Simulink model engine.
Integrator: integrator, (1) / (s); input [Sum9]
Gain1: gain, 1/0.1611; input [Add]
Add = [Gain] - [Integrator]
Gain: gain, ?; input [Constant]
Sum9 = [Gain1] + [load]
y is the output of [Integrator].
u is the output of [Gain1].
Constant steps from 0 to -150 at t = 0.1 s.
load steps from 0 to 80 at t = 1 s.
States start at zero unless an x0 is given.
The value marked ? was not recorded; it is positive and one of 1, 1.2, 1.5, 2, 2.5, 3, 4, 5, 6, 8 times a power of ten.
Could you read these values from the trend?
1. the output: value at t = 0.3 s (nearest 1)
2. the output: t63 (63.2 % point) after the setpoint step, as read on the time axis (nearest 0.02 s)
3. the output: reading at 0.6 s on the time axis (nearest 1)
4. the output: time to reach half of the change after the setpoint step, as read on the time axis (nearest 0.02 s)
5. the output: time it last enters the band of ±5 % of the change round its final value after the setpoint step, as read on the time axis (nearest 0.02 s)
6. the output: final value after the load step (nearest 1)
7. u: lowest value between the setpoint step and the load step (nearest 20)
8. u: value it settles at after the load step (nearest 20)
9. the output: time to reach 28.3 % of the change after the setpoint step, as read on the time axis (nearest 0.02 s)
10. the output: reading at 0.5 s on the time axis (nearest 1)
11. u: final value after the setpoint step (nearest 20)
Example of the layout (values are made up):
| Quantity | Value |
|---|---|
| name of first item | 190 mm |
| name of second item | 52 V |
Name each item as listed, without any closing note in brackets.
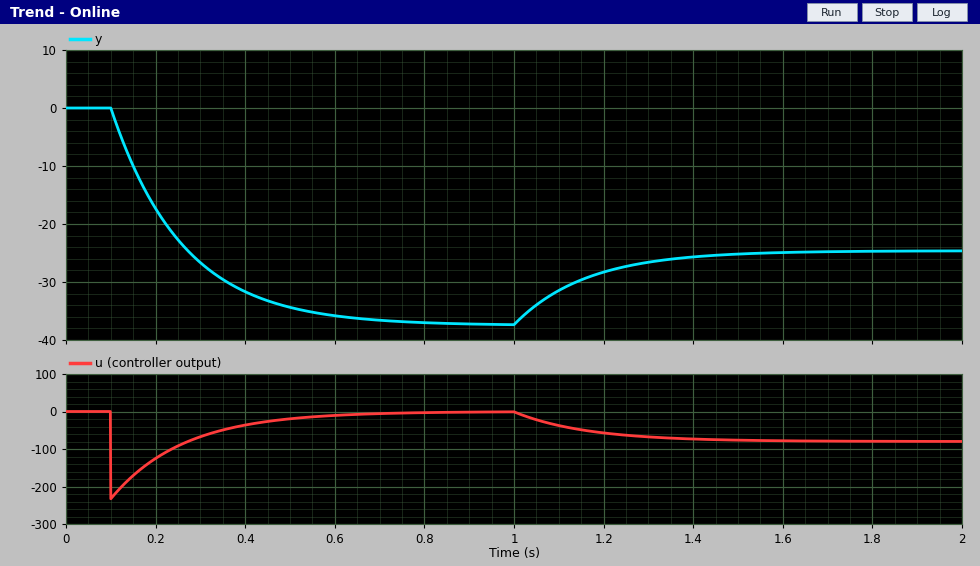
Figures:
| Quantity | Value |
|---|---|
| the output: value at t = 0.3 s | -27 |
| the output: t63 (63.2 % point) after the setpoint step, as read on the time axis | 0.26 s |
| the output: reading at 0.6 s on the time axis | -36 |
| the output: time to reach half of the change after the setpoint step, as read on the time axis | 0.22 s |
| the output: time it last enters the band of ±5 % of the change round its final value after the setpoint step, as read on the time axis | 0.58 s |
| the output: final value after the load step | -25 |
| u: lowest value between the setpoint step and the load step | -240 |
| u: value it settles at after the load step | -80 |
| the output: time to reach 28.3 % of the change after the setpoint step, as read on the time axis | 0.16 s |
| the output: reading at 0.5 s on the time axis | -34 |
| u: final value after the setpoint step | 0 |
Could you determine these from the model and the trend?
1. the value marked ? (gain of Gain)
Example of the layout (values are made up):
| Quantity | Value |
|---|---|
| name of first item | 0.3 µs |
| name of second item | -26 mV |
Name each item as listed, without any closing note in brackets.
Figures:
| Quantity | Value |
|---|---|
| the value marked ? | 0.25 |
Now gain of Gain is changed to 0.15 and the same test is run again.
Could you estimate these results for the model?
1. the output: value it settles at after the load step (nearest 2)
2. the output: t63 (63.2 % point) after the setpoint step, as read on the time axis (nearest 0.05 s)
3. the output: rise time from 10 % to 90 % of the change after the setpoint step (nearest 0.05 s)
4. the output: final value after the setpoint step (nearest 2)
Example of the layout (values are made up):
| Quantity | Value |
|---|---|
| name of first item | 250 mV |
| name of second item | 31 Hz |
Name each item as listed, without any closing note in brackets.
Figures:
| Quantity | Value |
|---|---|
| the output: value it settles at after the load step | -10 |
| the output: t63 (63.2 % point) after the setpoint step, as read on the time axis | 0.25 s |
| the output: rise time from 10 % to 90 % of the change after the setpoint step | 0.35 s |
| the output: final value after the setpoint step | -22 |
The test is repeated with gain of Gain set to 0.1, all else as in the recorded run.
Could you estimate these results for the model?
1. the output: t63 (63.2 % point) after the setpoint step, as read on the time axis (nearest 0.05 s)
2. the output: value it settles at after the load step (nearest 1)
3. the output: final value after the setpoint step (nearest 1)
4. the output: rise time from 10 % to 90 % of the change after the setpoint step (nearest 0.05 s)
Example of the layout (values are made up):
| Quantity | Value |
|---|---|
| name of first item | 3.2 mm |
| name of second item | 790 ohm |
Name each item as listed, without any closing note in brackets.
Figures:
| Quantity | Value |
|---|---|
| the output: t63 (63.2 % point) after the setpoint step, as read on the time axis | 0.25 s |
| the output: value it settles at after the load step | -2 |
| the output: final value after the setpoint step | -15 |
| the output: rise time from 10 % to 90 % of the change after the setpoint step | 0.35 s |
